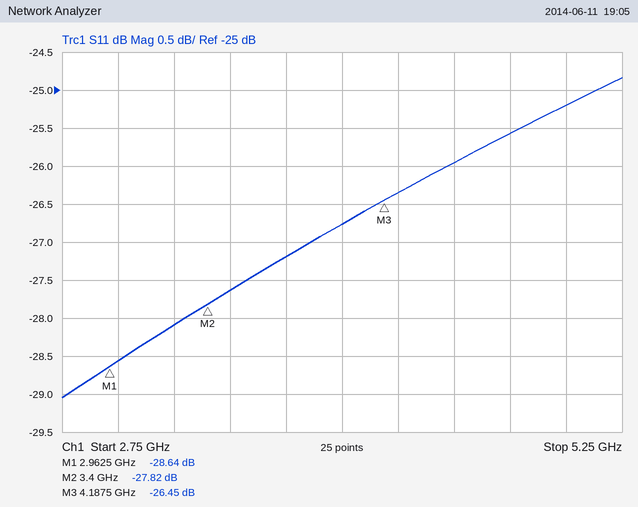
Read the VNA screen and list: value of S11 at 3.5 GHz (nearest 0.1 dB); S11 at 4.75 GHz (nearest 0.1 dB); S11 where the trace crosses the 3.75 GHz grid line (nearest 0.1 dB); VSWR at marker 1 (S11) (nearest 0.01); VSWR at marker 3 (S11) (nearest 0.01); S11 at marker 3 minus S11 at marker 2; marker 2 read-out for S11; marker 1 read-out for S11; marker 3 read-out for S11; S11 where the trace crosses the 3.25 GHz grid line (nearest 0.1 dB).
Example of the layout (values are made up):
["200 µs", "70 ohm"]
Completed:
["-27.6 dB", "-25.6 dB", "-27.2 dB", "1.08", "1.10", "1.37 dB", "-27.82 dB", "-28.64 dB", "-26.45 dB", "-28.1 dB"]
